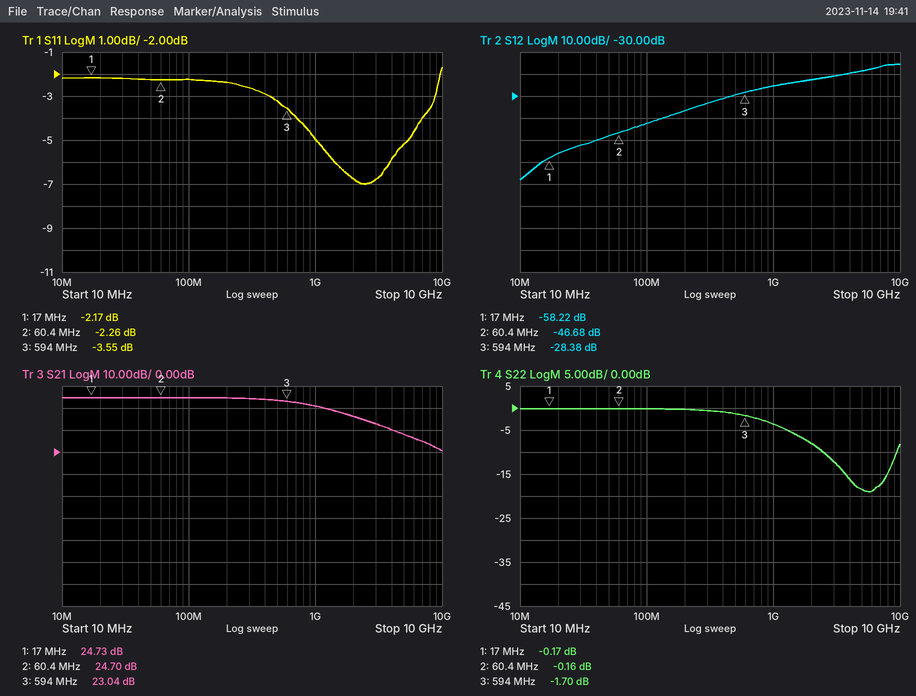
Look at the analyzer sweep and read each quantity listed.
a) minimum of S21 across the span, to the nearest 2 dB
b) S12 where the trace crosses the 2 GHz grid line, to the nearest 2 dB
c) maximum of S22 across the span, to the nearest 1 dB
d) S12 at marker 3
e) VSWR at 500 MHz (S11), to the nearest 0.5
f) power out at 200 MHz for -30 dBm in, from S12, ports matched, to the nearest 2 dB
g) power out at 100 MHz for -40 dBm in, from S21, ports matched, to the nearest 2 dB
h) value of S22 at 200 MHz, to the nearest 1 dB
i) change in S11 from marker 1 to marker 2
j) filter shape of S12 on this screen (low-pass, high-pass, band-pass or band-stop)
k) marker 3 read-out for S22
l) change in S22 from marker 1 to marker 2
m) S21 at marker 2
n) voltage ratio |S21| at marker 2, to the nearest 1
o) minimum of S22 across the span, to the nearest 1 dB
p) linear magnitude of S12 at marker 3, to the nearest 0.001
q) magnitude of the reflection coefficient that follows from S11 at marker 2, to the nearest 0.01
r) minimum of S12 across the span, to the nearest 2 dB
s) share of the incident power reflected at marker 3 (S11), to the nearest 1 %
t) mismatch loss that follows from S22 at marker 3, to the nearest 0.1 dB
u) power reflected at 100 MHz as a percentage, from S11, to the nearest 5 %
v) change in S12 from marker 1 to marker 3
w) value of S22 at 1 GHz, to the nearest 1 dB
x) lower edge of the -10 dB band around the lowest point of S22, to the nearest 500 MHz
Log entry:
0 dB
-22 dB
0 dB
-28.38 dB
5.5
-66 dBm
-16 dBm
0 dB
-0.09 dB
high-pass
-1.70 dB
0.01 dB
24.70 dB
17
-19 dB
0.038
0.77
-68 dB
44 %
4.9 dB
60 %
29.84 dB
-4 dB
2.5 GHz
